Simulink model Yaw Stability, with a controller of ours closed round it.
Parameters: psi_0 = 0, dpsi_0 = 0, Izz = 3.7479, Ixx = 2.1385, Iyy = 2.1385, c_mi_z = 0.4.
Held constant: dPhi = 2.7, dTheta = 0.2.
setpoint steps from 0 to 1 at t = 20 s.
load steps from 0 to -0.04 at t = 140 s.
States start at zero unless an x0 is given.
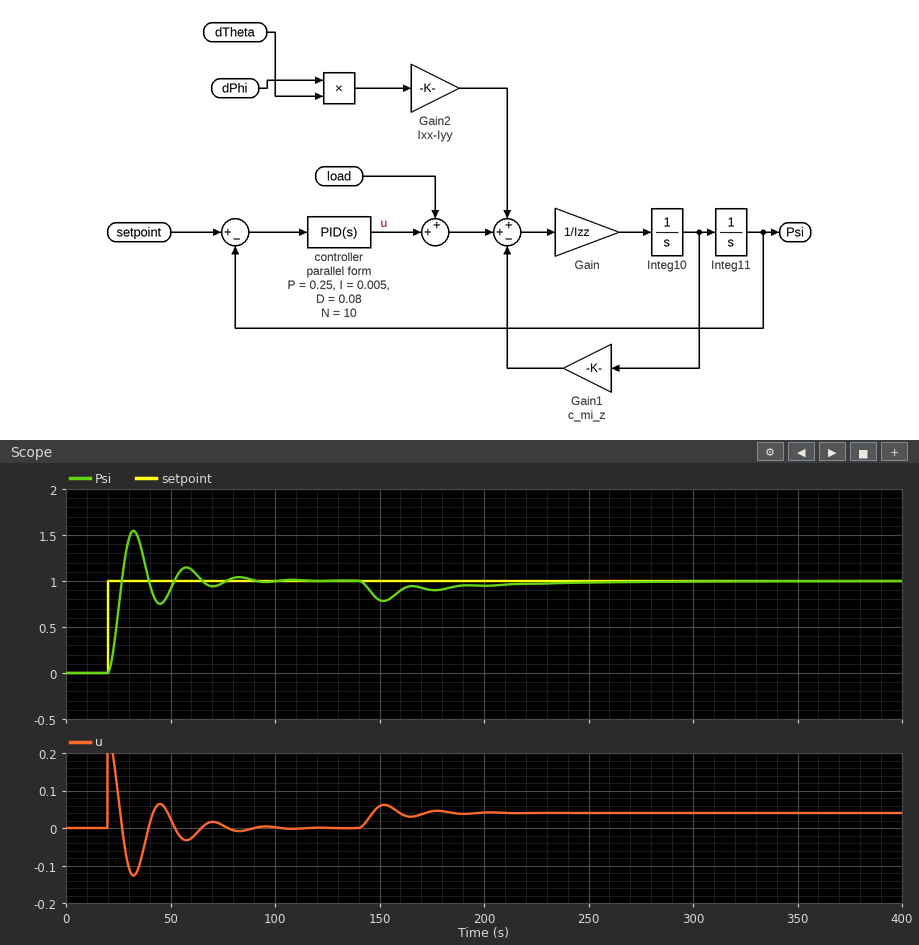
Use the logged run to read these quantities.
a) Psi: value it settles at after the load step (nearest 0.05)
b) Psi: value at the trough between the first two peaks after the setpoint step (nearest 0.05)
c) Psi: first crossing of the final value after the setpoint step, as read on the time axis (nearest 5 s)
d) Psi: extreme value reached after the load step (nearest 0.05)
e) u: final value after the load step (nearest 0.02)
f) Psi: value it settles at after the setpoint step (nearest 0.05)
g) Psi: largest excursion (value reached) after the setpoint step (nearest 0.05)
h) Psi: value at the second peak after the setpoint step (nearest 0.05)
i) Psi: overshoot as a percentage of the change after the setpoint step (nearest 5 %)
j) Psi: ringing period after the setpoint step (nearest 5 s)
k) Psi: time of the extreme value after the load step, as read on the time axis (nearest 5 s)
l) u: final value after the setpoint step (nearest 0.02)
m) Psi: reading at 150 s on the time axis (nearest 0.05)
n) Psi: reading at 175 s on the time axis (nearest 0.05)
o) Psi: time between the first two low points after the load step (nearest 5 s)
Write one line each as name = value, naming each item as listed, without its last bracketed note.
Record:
Psi: value it settles at after the load step = 1.00
Psi: value at the trough between the first two peaks after the setpoint step = 0.75
Psi: first crossing of the final value after the setpoint step, as read on the time axis = 25 s
Psi: extreme value reached after the load step = 0.80
u: final value after the load step = 0.04
Psi: value it settles at after the setpoint step = 1.00
Psi: largest excursion (value reached) after the setpoint step = 1.55
Psi: value at the second peak after the setpoint step = 1.15
Psi: overshoot as a percentage of the change after the setpoint step = 55 %
Psi: ringing period after the setpoint step = 25 s
Psi: time of the extreme value after the load step, as read on the time axis = 150 s
u: final value after the setpoint step = 0.00
Psi: reading at 150 s on the time axis = 0.80
Psi: reading at 175 s on the time axis = 0.90
Psi: time between the first two low points after the load step = 25 s
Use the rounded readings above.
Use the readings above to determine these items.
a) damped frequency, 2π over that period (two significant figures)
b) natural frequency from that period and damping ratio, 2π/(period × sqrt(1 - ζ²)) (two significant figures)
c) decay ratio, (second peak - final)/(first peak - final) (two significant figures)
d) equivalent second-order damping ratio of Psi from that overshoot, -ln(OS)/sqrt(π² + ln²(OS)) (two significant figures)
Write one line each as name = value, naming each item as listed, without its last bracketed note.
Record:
damped frequency, 2π over that period = 0.25 rad/s
natural frequency from that period and damping ratio, 2π/(period × sqrt(1 - ζ²)) = 0.26 rad/s
decay ratio, (second peak - final)/(first peak - final) = 0.27
equivalent second-order damping ratio of Psi from that overshoot, -ln(OS)/sqrt(π² + ln²(OS)) = 0.19
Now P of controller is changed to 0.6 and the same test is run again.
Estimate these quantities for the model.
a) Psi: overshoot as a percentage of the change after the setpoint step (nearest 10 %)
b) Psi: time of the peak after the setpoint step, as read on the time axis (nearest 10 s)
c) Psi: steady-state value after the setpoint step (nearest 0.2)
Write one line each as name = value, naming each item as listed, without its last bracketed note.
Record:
Psi: overshoot as a percentage of the change after the setpoint step = 60 %
Psi: time of the peak after the setpoint step, as read on the time axis = 30 s
Psi: steady-state value after the setpoint step = 1.0
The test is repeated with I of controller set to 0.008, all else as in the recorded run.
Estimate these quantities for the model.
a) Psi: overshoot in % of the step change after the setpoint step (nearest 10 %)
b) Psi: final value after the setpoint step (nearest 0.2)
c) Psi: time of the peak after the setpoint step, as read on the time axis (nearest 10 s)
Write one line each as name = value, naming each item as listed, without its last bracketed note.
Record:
Psi: overshoot in % of the step change after the setpoint step = 60 %
Psi: final value after the setpoint step = 1.0
Psi: time of the peak after the setpoint step, as read on the time axis = 30 s
